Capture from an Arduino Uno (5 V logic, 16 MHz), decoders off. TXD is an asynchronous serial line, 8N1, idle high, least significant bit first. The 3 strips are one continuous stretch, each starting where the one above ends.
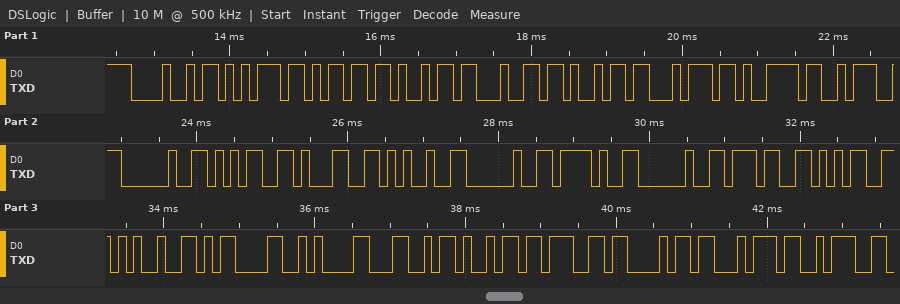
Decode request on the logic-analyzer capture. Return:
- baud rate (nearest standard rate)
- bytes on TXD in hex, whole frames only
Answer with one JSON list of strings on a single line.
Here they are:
["9600 baud", "48 75 6D 69 64 69 74 79 3A 20 35 31 25 20 2F 20 37 35 25 0D 0A 4C 69 67 68 74 3A"]
